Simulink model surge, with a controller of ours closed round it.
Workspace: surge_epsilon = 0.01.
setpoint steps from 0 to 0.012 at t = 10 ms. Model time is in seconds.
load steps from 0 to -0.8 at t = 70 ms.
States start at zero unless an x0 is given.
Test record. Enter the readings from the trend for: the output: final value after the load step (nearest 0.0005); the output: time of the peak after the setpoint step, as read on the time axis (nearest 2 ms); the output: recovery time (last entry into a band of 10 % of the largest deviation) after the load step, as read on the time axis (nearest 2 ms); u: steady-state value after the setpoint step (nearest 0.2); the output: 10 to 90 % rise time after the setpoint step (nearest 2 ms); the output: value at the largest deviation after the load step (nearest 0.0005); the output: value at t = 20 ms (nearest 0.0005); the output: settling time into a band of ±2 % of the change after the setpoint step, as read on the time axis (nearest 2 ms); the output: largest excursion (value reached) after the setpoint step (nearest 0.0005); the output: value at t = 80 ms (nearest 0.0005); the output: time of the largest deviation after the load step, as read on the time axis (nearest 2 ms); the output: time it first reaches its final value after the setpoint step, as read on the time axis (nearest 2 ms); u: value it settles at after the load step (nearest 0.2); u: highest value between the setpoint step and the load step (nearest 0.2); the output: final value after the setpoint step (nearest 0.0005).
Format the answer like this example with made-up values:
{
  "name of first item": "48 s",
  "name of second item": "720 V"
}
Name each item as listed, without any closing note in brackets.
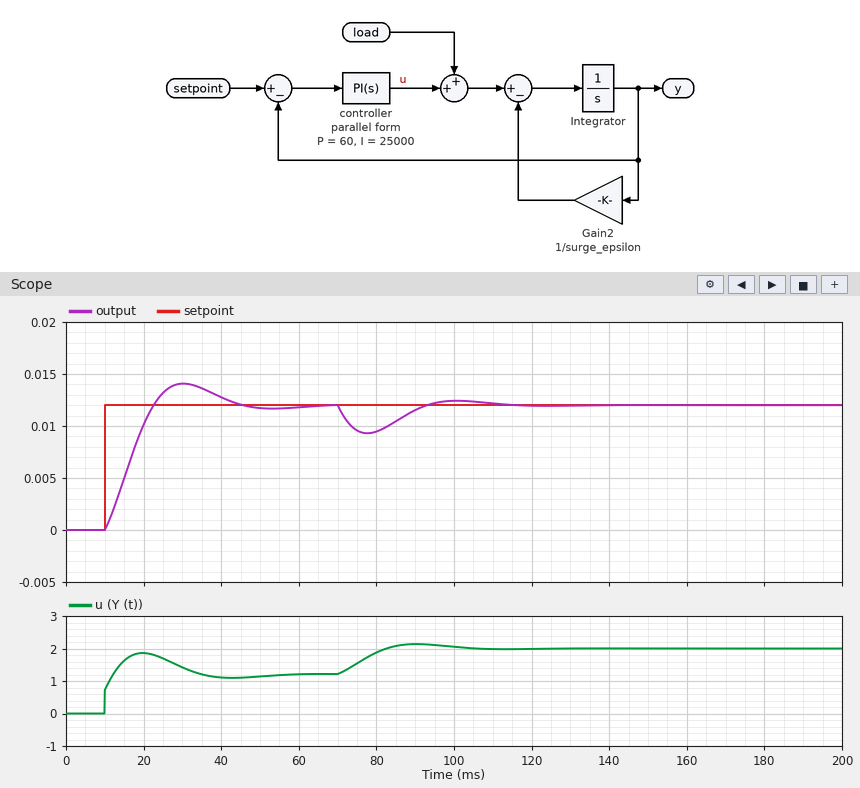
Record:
{
  "the output: final value after the load step": "0.0120",
  "the output: time of the peak after the setpoint step, as read on the time axis": "30 ms",
  "the output: recovery time (last entry into a band of 10 % of the largest deviation) after the load step, as read on the time axis": "108 ms",
  "u: steady-state value after the setpoint step": "1.2",
  "the output: 10 to 90 % rise time after the setpoint step": "10 ms",
  "the output: value at the largest deviation after the load step": "0.0095",
  "the output: value at t = 20 ms": "0.0100",
  "the output: settling time into a band of ±2 % of the change after the setpoint step, as read on the time axis": "58 ms",
  "the output: largest excursion (value reached) after the setpoint step": "0.0140",
  "the output: value at t = 80 ms": "0.0095",
  "the output: time of the largest deviation after the load step, as read on the time axis": "78 ms",
  "the output: time it first reaches its final value after the setpoint step, as read on the time axis": "22 ms",
  "u: value it settles at after the load step": "2.0",
  "u: highest value between the setpoint step and the load step": "1.8",
  "the output: final value after the setpoint step": "0.0120"
}
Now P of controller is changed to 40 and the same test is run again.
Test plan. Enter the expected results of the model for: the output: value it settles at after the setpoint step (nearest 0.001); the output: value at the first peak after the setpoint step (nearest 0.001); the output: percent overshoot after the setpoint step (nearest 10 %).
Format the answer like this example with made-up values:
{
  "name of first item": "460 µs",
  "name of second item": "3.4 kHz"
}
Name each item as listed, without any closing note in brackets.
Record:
{
  "the output: value it settles at after the setpoint step": "0.012",
  "the output: value at the first peak after the setpoint step": "0.015",
  "the output: percent overshoot after the setpoint step": "20 %"
}
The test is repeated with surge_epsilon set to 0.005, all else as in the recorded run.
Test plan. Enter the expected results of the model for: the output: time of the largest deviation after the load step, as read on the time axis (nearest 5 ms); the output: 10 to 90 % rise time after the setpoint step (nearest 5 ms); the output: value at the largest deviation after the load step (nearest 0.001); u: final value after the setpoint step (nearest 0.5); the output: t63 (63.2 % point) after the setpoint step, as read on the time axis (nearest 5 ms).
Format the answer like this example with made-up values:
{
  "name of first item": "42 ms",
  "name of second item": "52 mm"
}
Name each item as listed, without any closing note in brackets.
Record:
{
  "the output: time of the largest deviation after the load step, as read on the time axis": "75 ms",
  "the output: 10 to 90 % rise time after the setpoint step": "15 ms",
  "the output: value at the largest deviation after the load step": "0.010",
  "u: final value after the setpoint step": "2.5",
  "the output: t63 (63.2 % point) after the setpoint step, as read on the time axis": "20 ms"
}
